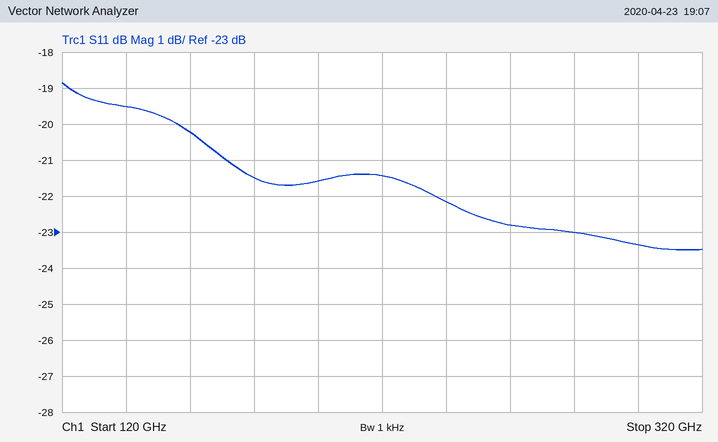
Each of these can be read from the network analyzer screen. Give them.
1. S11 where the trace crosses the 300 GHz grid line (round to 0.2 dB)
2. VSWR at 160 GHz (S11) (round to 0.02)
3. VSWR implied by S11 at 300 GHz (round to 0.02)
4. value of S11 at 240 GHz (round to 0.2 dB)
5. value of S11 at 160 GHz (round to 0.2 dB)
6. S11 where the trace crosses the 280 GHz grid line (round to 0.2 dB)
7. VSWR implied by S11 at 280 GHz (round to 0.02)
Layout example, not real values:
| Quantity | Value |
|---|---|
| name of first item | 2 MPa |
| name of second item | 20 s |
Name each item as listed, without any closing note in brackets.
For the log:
| Quantity | Value |
|---|---|
| S11 where the trace crosses the 300 GHz grid line | -23.4 dB |
| VSWR at 160 GHz (S11) | 1.22 |
| VSWR implied by S11 at 300 GHz | 1.14 |
| value of S11 at 240 GHz | -22.2 dB |
| value of S11 at 160 GHz | -20.2 dB |
| S11 where the trace crosses the 280 GHz grid line | -23.0 dB |
| VSWR implied by S11 at 280 GHz | 1.16 |
